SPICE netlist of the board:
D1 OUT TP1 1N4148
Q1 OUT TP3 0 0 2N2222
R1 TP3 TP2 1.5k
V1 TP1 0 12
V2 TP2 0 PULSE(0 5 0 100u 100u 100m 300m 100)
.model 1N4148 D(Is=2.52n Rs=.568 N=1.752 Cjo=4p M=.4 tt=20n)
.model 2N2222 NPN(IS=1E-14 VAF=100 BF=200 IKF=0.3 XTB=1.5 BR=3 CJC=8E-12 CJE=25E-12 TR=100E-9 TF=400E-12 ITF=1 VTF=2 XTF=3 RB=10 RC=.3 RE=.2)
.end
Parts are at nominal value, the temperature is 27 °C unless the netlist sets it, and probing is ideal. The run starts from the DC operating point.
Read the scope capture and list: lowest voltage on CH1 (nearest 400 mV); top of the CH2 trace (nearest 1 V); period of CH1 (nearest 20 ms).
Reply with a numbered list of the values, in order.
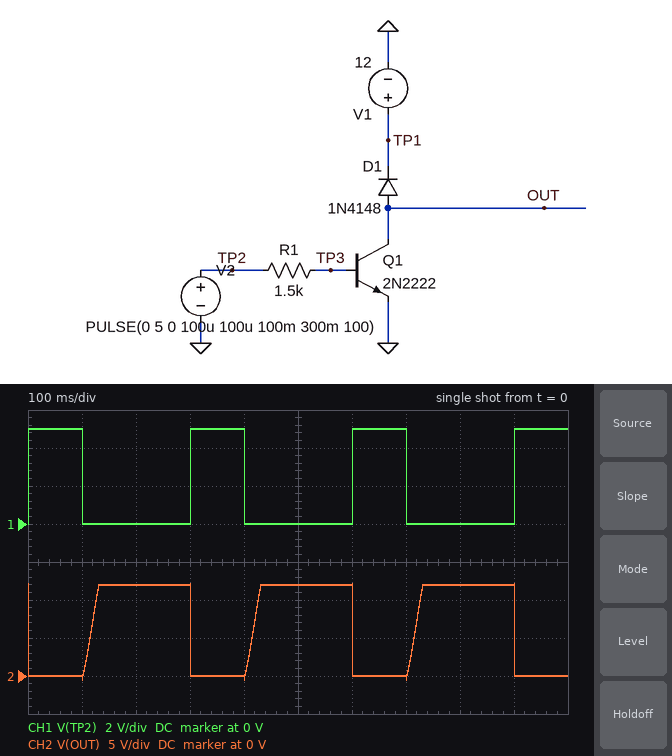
1. 0 V
2. 12 V
3. 300 ms
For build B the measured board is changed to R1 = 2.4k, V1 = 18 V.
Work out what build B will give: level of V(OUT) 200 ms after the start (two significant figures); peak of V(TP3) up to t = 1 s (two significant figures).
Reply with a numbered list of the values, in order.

1. 18 V
2. 720 mV
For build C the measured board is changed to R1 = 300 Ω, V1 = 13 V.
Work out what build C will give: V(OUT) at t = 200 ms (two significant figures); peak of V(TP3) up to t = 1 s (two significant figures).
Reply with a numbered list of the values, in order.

1. 13 V
2. 900 mV
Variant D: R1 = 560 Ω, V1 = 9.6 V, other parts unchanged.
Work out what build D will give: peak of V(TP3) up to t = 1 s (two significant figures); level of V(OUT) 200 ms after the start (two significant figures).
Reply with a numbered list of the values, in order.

1. 820 mV
2. 9.6 V
